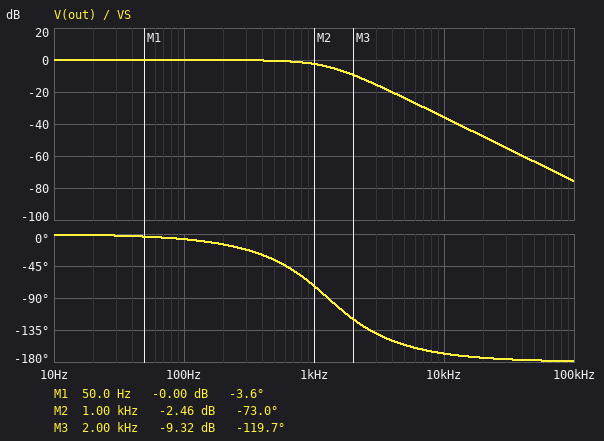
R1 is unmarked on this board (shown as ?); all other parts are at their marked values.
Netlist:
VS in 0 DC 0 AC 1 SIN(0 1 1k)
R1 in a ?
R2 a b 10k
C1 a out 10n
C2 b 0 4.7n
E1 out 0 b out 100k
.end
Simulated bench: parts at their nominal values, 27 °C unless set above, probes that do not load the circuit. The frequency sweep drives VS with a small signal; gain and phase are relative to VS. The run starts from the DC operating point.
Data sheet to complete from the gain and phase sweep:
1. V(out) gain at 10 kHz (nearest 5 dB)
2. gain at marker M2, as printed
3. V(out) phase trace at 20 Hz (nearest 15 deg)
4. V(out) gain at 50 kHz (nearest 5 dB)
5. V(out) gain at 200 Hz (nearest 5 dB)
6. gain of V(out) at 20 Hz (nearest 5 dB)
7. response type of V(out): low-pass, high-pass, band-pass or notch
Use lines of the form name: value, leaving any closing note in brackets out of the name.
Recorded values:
V(out) gain at 10 kHz: -35 dB
gain at marker M2, as printed: -2.46 dB
V(out) phase trace at 20 Hz: 0 deg
V(out) gain at 50 kHz: -65 dB
V(out) gain at 200 Hz: 0 dB
gain of V(out) at 20 Hz: 0 dB
response type of V(out): low-pass, high-pass, band-pass or notch: low-pass
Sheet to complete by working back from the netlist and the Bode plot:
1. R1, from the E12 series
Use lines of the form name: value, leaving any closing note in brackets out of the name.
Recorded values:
R1, from the E12 series: 33 kΩ
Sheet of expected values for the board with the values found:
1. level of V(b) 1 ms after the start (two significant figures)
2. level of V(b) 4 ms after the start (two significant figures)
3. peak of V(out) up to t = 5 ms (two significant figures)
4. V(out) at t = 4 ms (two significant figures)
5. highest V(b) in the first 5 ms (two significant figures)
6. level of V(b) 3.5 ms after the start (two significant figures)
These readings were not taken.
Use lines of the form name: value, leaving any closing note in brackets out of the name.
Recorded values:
level of V(b) 1 ms after the start: -720 mV
level of V(b) 4 ms after the start: -720 mV
peak of V(out) up to t = 5 ms: 770 mV
V(out) at t = 4 ms: -720 mV
highest V(b) in the first 5 ms: 770 mV
level of V(b) 3.5 ms after the start: 720 mV
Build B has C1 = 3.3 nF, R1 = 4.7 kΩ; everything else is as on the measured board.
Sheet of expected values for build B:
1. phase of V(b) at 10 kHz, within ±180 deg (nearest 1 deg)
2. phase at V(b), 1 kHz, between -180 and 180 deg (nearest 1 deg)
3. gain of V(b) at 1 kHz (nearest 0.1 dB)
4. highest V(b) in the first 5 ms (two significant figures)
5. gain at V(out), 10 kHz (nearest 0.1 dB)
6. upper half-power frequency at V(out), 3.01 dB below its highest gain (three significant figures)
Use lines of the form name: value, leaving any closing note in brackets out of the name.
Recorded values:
phase of V(b) at 10 kHz, within ±180 deg: -113 deg
phase at V(b), 1 kHz, between -180 and 180 deg: -24 deg
gain of V(b) at 1 kHz: -0.5 dB
highest V(b) in the first 5 ms: 940 mV
gain at V(out), 10 kHz: -13.5 dB
upper half-power frequency at V(out), 3.01 dB below its highest gain: 2.70 kHz
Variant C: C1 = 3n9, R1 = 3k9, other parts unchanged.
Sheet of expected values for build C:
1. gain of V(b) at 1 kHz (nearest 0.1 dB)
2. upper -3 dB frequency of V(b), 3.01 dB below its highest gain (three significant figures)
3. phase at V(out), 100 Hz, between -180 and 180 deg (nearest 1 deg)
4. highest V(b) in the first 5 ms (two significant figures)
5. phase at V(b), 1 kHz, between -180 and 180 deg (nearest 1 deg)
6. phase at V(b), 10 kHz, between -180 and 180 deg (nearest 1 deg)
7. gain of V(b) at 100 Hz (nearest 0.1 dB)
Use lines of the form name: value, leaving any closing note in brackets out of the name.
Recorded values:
gain of V(b) at 1 kHz: -0.5 dB
upper -3 dB frequency of V(b), 3.01 dB below its highest gain: 2.90 kHz
phase at V(out), 100 Hz, between -180 and 180 deg: -2 deg
highest V(b) in the first 5 ms: 950 mV
phase at V(b), 1 kHz, between -180 and 180 deg: -23 deg
phase at V(b), 10 kHz, between -180 and 180 deg: -114 deg
gain of V(b) at 100 Hz: 0 dB
